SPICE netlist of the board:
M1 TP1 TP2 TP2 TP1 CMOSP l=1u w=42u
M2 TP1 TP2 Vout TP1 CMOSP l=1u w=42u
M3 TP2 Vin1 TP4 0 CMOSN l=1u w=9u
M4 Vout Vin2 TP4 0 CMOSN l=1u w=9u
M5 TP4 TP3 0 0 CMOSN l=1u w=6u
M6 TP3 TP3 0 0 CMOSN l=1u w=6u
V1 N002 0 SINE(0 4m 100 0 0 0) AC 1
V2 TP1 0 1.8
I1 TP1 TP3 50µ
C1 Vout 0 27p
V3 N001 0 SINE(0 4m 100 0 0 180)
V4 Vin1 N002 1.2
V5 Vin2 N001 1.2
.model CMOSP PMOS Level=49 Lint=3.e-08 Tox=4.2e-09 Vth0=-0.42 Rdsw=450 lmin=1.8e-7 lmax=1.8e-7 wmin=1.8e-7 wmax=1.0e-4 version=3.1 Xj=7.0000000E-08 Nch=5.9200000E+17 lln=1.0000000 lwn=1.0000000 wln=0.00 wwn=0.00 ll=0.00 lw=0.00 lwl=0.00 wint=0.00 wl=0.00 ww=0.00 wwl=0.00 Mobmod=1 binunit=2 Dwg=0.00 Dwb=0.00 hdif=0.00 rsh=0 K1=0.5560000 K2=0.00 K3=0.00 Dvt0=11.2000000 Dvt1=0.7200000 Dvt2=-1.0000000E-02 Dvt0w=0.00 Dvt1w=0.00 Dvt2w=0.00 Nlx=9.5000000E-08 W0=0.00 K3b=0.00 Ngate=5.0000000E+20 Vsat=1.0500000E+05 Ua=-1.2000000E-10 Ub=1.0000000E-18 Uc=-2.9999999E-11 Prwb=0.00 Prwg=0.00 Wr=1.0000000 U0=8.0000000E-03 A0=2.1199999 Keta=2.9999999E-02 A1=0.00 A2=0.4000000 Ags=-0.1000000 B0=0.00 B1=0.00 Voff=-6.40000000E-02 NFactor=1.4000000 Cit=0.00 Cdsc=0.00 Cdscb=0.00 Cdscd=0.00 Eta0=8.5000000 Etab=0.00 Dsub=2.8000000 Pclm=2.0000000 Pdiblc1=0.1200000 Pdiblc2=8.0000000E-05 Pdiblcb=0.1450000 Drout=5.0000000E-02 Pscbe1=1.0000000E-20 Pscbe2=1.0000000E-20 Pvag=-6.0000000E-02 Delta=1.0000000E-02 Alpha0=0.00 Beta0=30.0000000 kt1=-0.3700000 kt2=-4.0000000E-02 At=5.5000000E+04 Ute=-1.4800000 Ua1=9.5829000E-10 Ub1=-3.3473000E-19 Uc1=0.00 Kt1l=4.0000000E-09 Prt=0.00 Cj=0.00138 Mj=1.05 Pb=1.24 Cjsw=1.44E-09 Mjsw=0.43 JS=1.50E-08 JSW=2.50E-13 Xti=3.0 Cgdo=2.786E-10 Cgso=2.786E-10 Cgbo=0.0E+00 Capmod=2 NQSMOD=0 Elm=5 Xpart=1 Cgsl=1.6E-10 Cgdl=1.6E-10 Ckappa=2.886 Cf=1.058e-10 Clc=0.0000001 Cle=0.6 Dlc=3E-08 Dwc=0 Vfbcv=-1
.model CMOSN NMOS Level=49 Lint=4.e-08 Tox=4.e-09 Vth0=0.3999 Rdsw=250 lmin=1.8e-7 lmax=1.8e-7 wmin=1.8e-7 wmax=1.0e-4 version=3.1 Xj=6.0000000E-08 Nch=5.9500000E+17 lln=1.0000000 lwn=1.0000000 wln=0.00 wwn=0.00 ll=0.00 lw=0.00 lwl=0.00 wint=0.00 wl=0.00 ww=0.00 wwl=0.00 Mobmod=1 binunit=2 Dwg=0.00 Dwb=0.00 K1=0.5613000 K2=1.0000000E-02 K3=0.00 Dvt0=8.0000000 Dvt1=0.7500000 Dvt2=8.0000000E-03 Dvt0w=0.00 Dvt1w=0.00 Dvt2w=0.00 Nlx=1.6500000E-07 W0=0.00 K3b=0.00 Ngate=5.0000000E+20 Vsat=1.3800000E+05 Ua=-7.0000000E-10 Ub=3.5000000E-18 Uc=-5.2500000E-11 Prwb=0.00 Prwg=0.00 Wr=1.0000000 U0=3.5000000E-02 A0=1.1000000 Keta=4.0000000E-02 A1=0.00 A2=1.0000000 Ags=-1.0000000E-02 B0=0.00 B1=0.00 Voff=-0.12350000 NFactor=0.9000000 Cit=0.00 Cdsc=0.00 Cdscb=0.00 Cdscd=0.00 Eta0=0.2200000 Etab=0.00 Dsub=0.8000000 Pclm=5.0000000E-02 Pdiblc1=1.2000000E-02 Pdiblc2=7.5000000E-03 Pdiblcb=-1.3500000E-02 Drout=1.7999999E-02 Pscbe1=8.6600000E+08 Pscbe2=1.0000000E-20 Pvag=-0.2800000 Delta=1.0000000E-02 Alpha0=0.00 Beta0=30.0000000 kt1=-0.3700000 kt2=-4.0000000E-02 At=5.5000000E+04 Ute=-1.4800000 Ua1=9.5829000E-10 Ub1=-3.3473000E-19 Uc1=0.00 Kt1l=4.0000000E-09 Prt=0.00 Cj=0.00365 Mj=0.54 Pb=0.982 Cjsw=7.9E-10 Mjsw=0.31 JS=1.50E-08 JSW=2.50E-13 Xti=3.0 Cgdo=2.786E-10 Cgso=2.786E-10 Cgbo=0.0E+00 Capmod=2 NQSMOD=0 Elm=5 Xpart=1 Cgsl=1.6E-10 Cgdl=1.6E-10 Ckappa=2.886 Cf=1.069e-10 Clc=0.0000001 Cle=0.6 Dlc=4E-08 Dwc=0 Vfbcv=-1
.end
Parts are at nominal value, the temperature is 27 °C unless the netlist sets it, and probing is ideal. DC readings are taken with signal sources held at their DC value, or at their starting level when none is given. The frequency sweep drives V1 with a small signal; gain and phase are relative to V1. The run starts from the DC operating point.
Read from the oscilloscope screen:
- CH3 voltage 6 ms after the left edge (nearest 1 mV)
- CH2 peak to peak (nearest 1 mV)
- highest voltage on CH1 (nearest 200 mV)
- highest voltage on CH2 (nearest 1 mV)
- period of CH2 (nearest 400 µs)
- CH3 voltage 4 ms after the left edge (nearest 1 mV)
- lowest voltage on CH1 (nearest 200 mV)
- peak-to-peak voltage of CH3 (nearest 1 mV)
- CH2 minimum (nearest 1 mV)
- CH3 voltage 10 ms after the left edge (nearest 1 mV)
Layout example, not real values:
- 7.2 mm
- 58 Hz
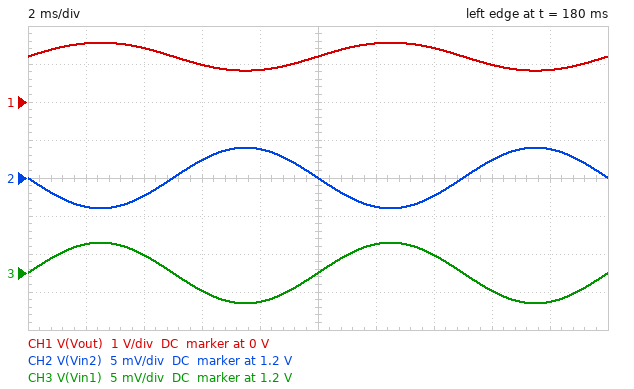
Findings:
- 1.198 V
- 8 mV
- 1.6 V
- 1.204 V
- 10.0 ms
- 1.202 V
- 800 mV
- 8 mV
- 1.196 V
- 1.200 V
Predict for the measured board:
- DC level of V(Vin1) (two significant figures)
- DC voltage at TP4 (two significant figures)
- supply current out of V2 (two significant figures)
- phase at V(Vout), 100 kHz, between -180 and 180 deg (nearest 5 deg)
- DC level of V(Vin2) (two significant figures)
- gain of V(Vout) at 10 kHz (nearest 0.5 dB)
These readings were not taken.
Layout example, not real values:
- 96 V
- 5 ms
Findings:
- 1.2 V
- 490 mV
- 99 µA
- -70 deg
- 1.2 V
- 33.0 dB
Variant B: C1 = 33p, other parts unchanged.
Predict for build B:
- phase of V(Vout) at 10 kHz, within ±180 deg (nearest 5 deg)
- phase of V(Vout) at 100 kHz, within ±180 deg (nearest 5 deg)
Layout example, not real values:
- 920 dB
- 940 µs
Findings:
- -20 deg
- -75 deg
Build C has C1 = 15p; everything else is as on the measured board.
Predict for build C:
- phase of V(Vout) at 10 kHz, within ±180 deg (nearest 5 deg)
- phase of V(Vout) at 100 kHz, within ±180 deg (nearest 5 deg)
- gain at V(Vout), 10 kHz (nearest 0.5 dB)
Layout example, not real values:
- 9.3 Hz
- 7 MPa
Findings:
- -10 deg
- -60 deg
- 33.5 dB
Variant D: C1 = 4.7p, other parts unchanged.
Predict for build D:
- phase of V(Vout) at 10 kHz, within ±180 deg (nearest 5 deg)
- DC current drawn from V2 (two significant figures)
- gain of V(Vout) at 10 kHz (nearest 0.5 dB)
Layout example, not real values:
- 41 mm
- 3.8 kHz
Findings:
- -5 deg
- 99 µA
- 33.5 dB
